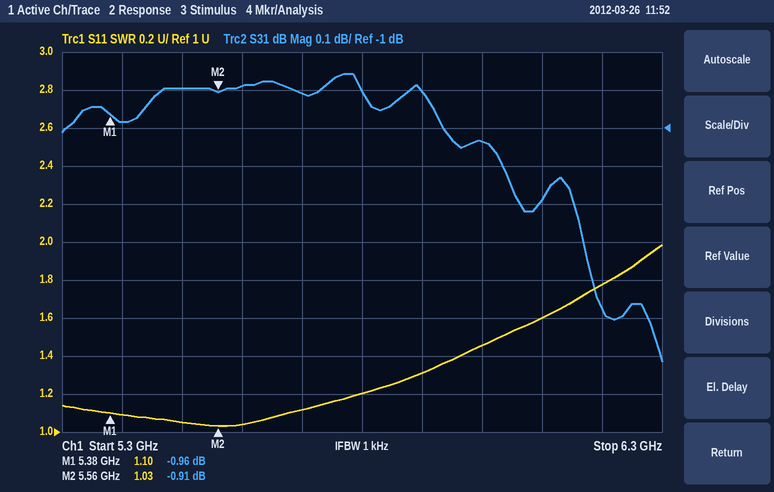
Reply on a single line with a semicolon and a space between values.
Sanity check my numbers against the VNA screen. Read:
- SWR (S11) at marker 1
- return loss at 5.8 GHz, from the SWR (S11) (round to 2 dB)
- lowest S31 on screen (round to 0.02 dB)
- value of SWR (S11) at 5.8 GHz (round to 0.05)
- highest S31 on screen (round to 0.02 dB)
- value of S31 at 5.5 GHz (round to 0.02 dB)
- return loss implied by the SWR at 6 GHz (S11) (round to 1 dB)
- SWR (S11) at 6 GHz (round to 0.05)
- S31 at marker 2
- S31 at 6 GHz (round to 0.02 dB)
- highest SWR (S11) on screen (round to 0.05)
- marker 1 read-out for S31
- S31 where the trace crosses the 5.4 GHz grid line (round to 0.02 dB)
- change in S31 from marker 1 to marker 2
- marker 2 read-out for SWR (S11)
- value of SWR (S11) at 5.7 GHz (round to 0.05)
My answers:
1.10; 20 dB; -1.62 dB; 1.20; -0.86 dB; -0.90 dB; 15 dB; 1.45; -0.91 dB; -1.04 dB; 2.00; -0.96 dB; -0.98 dB; 0.05 dB; 1.03; 1.10
